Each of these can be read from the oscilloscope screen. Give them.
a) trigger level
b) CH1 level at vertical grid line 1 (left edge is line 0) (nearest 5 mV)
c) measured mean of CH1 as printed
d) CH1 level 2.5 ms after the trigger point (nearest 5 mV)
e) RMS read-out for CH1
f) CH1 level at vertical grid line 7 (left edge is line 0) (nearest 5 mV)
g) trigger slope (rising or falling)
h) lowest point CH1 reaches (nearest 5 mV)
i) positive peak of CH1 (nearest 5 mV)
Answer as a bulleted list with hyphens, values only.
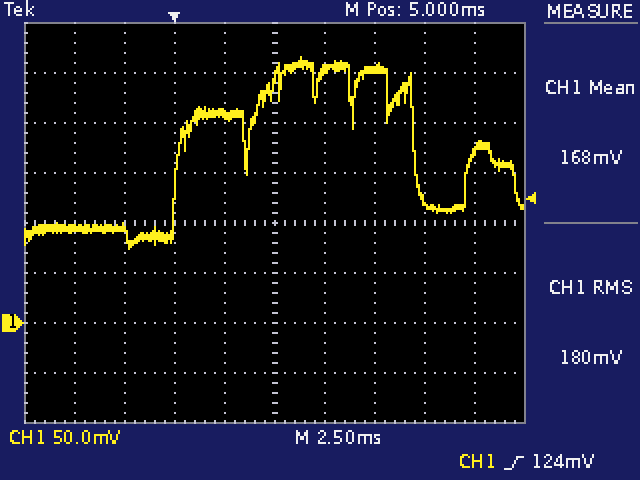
- 124 mV
- 95 mV
- 168 mV
- 210 mV
- 180 mV
- 255 mV
- rising
- 75 mV
- 265 mV
